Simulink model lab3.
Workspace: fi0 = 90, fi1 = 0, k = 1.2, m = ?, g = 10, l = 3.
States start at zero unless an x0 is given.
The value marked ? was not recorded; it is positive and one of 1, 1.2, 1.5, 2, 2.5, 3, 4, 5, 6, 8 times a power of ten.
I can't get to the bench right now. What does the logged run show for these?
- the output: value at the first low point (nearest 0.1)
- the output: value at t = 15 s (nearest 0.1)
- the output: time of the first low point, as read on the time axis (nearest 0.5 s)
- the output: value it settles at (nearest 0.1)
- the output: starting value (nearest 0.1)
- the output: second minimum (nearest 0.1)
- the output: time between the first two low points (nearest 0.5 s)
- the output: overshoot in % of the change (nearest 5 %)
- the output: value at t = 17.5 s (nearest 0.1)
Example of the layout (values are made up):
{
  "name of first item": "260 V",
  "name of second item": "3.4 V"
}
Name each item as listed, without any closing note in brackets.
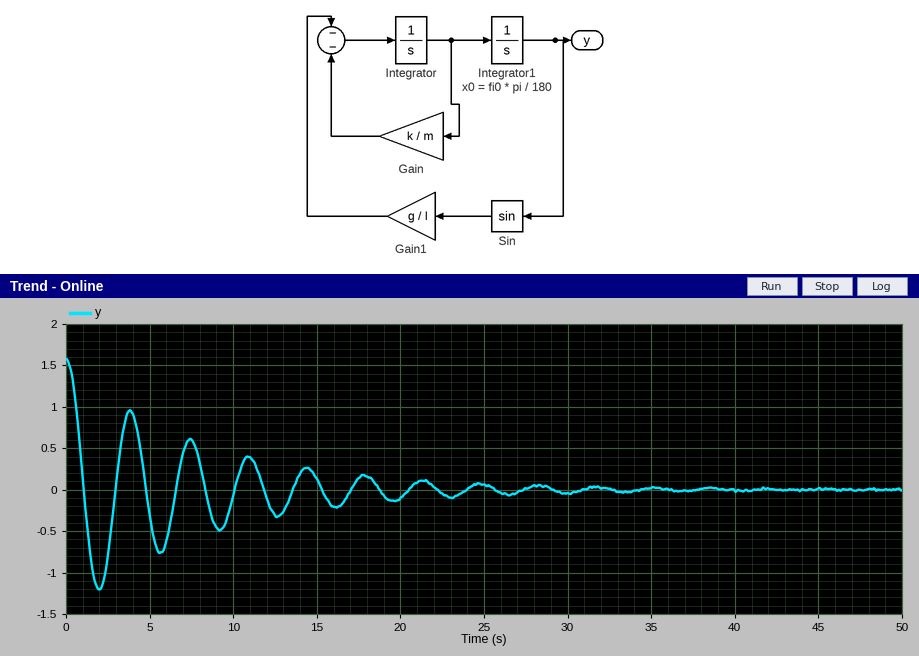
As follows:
{
  "the output: value at the first low point": "-1.2",
  "the output: value at t = 15 s": "0.1",
  "the output: time of the first low point, as read on the time axis": "2.0 s",
  "the output: value it settles at": "0.0",
  "the output: starting value": "1.6",
  "the output: second minimum": "-0.8",
  "the output: time between the first two low points": "3.5 s",
  "the output: overshoot in % of the change": "75 %",
  "the output: value at t = 17.5 s": "0.1"
}
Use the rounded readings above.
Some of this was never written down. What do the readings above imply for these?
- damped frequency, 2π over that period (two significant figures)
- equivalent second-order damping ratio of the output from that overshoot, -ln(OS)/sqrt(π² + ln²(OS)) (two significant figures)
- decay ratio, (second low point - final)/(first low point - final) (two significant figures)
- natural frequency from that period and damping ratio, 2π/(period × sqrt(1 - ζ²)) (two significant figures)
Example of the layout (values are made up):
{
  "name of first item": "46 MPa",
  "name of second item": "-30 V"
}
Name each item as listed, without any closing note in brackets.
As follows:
{
  "damped frequency, 2π over that period": "1.8 rad/s",
  "equivalent second-order damping ratio of the output from that overshoot, -ln(OS)/sqrt(π² + ln²(OS))": "0.091",
  "decay ratio, (second low point - final)/(first low point - final)": "0.67",
  "natural frequency from that period and damping ratio, 2π/(period × sqrt(1 - ζ²))": "1.8 rad/s"
}
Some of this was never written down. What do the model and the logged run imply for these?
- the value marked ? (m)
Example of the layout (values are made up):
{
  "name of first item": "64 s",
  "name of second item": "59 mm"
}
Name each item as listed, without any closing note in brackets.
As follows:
{
  "the value marked ?": "5"
}
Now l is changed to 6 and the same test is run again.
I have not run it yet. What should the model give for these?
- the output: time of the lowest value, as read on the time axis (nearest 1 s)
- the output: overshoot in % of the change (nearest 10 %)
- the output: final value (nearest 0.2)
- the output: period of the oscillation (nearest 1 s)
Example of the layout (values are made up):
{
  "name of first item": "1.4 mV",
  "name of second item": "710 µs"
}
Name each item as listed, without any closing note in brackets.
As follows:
{
  "the output: time of the lowest value, as read on the time axis": "3 s",
  "the output: overshoot in % of the change": "70 %",
  "the output: final value": "0.0",
  "the output: period of the oscillation": "5 s"
}
